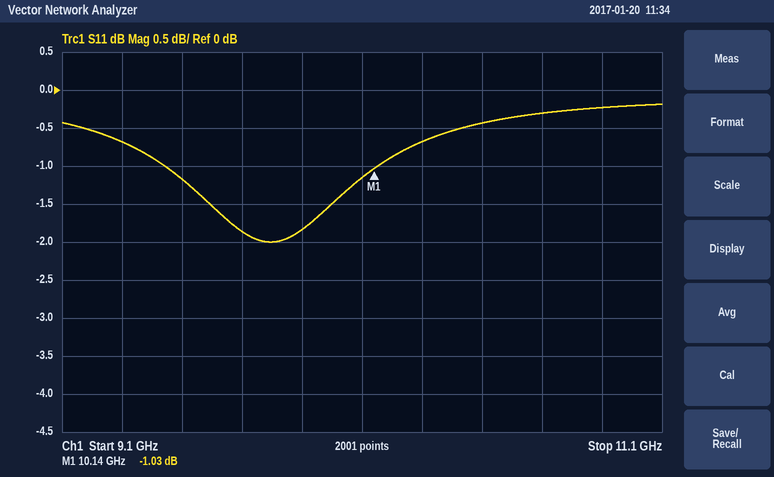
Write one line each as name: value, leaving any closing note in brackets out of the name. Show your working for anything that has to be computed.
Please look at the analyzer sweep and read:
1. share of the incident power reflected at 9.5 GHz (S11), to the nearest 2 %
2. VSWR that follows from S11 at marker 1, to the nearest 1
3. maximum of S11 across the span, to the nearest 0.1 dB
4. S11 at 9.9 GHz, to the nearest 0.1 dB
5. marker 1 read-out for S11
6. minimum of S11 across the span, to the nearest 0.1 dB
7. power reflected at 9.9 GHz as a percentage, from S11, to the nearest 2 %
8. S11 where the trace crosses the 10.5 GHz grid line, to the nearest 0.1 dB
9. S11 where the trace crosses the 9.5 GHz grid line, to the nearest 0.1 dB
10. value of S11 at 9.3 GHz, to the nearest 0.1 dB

share of the incident power reflected at 9.5 GHz (S11), to the nearest 2 %: 10^(-1.2/10) ≈ 76 %
VSWR that follows from S11 at marker 1, to the nearest 1: (1 + 0.8882)/(1 − 0.8882) ≈ 17
maximum of S11 across the span, to the nearest 0.1 dB: -0.2 dB
S11 at 9.9 GHz, to the nearest 0.1 dB: -1.8 dB
marker 1 read-out for S11: -1.03 dB
minimum of S11 across the span, to the nearest 0.1 dB: -2.0 dB
power reflected at 9.9 GHz as a percentage, from S11, to the nearest 2 %: 10^(-1.8/10) ≈ 66 %
S11 where the trace crosses the 10.5 GHz grid line, to the nearest 0.1 dB: -0.4 dB
S11 where the trace crosses the 9.5 GHz grid line, to the nearest 0.1 dB: -1.2 dB
value of S11 at 9.3 GHz, to the nearest 0.1 dB: -0.7 dB
